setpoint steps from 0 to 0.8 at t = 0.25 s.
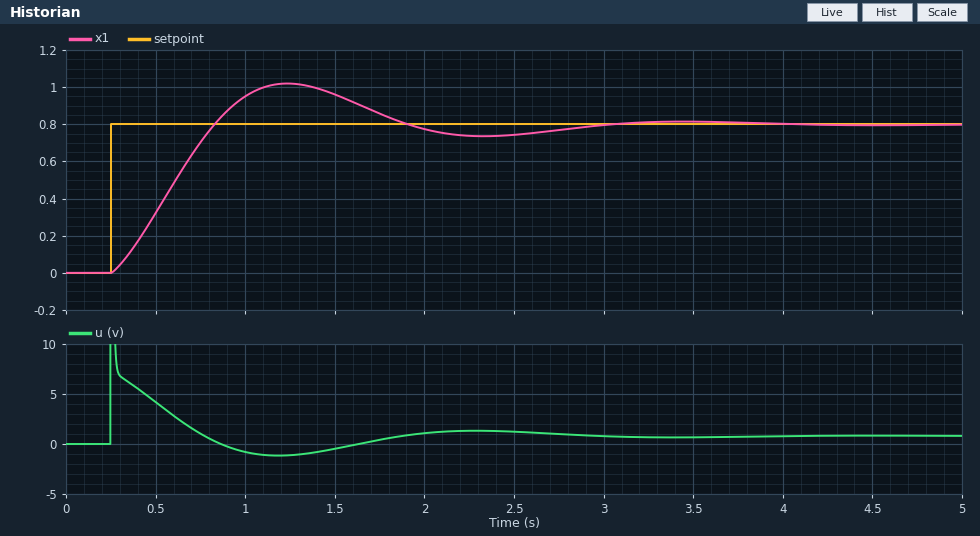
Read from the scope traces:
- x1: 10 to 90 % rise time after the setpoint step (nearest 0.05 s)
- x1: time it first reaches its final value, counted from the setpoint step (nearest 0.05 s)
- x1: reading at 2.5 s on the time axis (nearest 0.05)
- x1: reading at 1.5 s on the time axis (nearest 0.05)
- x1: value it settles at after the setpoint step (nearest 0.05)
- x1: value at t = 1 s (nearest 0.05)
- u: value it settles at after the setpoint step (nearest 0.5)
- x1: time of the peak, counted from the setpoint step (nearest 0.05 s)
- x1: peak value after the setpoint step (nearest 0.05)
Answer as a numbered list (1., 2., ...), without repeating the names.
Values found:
1. 0.45 s
2. 0.60 s
3. 0.75
4. 0.95
5. 0.80
6. 0.95
7. 1.0
8. 1.00 s
9. 1.00
